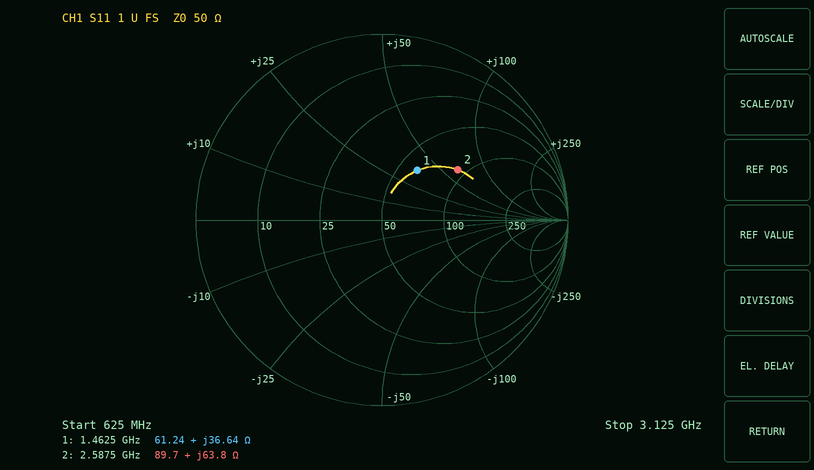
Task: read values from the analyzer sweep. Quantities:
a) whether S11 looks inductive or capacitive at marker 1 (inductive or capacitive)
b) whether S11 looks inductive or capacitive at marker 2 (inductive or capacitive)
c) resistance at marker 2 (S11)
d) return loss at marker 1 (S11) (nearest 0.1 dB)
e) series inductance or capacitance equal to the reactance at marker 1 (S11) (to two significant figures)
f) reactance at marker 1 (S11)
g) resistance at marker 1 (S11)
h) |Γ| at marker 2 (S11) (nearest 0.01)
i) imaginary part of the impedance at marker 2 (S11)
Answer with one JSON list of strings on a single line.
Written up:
["inductive", "inductive", "89.7 Ω", "9.7 dB", "4.0 nH", "+36.64 Ω", "61.24 Ω", "0.49", "+63.8 Ω"]
